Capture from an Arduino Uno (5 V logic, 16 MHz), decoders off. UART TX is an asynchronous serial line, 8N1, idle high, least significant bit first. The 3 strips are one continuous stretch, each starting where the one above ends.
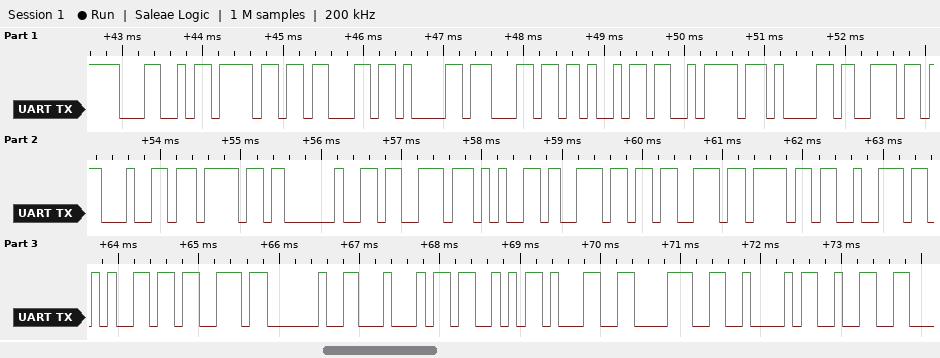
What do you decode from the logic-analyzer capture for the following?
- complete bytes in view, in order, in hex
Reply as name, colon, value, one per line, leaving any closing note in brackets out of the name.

complete bytes in view, in order, in hex: 0x4C 0x6F 0x63 0x61 0x6C 0x69 0x7A 0x61 0x6E 0x64 0x6F 0x20 0x73 0x65 0x6E 0x73 0x6F 0x72 0x65 0x73 0x20 0x44 0x53 0x31 0x38 0x42 0x32
